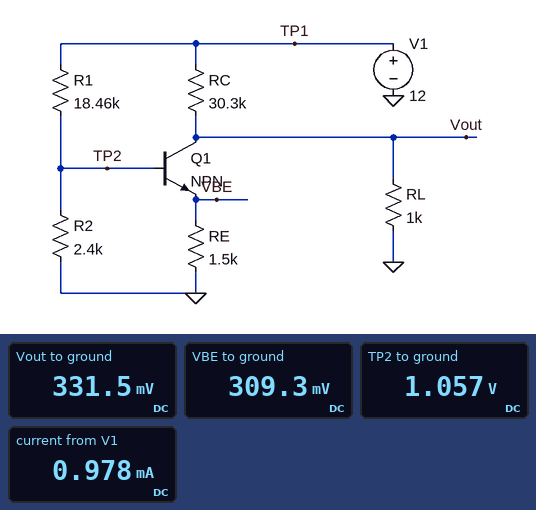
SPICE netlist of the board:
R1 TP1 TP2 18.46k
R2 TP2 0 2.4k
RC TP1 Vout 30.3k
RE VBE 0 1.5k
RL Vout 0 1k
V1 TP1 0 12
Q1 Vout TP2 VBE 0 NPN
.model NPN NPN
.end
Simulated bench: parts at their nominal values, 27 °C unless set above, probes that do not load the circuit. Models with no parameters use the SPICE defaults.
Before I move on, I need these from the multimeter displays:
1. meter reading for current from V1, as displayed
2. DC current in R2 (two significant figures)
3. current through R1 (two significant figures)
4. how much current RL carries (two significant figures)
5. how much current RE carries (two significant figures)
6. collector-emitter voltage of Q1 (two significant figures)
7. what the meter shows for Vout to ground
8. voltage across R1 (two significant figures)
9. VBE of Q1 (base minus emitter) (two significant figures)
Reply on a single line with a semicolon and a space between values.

0.978 mA; 440 µA; 590 µA; 330 µA; 210 µA; 22 mV; 331.5 mV; 11 V; 750 mV
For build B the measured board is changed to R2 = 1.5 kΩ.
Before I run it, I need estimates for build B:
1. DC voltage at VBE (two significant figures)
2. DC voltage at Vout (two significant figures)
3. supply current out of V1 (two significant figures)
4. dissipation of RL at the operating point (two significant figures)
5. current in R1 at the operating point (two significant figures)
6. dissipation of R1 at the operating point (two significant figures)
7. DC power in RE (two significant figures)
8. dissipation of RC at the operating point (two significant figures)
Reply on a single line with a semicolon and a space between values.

180 mV; 270 mV; 990 µA; 75 µW; 600 µA; 6.7 mW; 21 µW; 4.5 mW
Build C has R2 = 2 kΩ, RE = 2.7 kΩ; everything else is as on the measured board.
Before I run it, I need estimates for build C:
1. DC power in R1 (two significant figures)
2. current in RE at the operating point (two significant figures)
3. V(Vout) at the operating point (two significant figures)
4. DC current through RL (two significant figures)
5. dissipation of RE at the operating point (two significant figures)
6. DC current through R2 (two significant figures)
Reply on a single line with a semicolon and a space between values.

6.5 mW; 120 µA; 340 mV; 340 µA; 37 µW; 520 µA
